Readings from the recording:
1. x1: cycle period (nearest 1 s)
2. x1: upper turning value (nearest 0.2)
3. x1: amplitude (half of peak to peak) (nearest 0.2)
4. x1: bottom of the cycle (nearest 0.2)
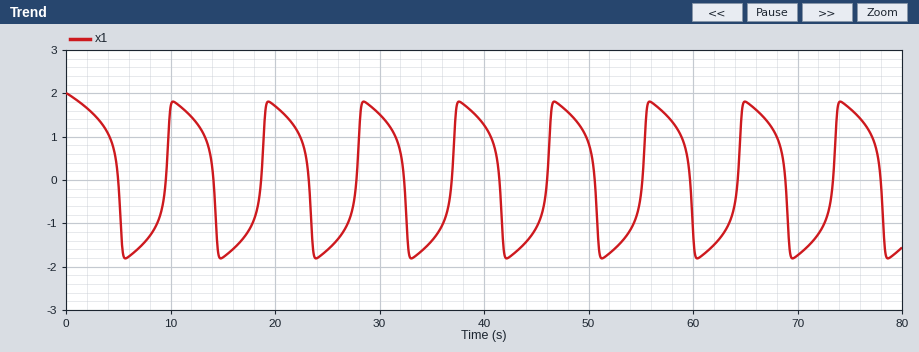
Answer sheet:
9 s
1.8
1.8
-1.8
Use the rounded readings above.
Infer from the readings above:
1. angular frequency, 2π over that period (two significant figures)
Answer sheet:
0.70 rad/s
